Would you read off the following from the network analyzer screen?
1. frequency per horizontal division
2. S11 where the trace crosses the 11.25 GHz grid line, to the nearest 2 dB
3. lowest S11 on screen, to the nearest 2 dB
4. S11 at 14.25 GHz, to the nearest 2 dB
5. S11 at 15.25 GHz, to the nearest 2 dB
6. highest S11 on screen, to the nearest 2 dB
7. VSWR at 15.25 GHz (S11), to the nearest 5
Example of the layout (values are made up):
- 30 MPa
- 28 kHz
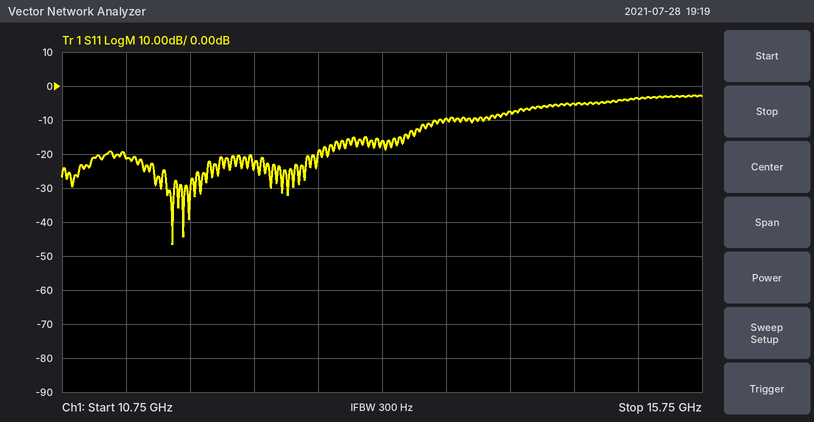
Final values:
- 500 MHz
- -22 dB
- -46 dB
- -8 dB
- -4 dB
- -2 dB
- 5
